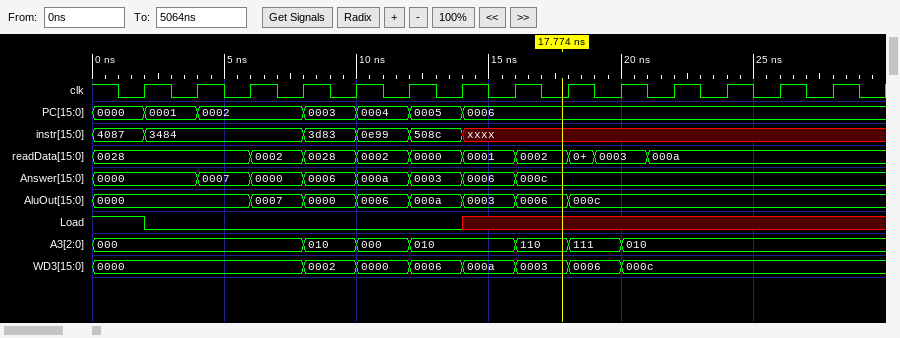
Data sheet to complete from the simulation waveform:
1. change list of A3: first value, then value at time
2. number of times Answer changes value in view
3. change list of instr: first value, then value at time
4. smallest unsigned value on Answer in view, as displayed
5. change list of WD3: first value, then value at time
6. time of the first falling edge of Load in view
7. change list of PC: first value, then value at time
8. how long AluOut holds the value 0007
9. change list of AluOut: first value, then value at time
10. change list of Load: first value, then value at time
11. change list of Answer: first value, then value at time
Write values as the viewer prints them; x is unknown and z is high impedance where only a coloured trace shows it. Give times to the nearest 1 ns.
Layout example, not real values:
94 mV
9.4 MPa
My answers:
000, 010 at 8 ns, 000 at 10 ns, 010 at 12 ns, 110 at 16 ns, 111 at 18 ns, 010 at 20 ns
7
4087, 3484 at 2 ns, 3d83 at 8 ns, 0e99 at 10 ns, 508c at 12 ns, xxxx at 14 ns
0000
0000, 0002 at 8 ns, 0000 at 10 ns, 0006 at 12 ns, 000a at 14 ns, 0003 at 16 ns, 0006 at 18 ns, 000c at 20 ns
2 ns
0000, 0001 at 2 ns, 0002 at 4 ns, 0003 at 8 ns, 0004 at 10 ns, 0005 at 12 ns, 0006 at 14 ns
2 ns
0000, 0007 at 6 ns, 0000 at 8 ns, 0006 at 10 ns, 000a at 12 ns, 0003 at 14 ns, 0006 at 16 ns, 000c at 18 ns
1, 0 at 2 ns, x at 14 ns
0000, 0007 at 4 ns, 0000 at 6 ns, 0006 at 8 ns, 000a at 10 ns, 0003 at 12 ns, 0006 at 14 ns, 000c at 16 ns
